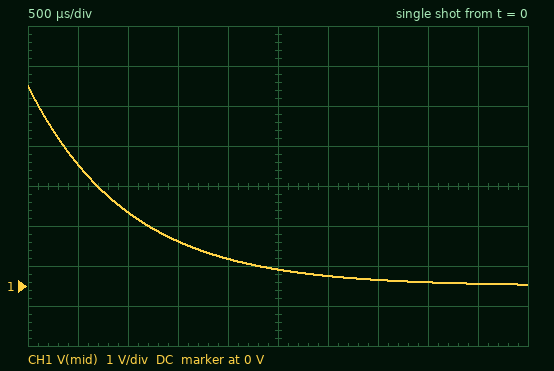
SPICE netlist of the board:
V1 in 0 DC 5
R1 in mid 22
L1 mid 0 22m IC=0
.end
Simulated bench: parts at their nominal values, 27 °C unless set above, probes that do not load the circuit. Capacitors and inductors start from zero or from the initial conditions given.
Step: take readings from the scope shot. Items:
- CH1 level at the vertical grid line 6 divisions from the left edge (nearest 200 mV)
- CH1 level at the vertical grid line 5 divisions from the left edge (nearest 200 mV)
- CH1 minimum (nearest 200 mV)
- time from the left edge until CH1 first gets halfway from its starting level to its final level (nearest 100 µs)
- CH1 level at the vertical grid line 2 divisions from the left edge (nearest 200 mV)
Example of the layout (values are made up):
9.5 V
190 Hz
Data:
200 mV
400 mV
0 V
700 µs
1.8 V
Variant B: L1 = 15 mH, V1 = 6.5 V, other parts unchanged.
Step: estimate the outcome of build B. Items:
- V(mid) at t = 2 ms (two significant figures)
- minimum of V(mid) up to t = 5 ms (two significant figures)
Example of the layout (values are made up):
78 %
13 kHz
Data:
350 mV
4.2 mV
